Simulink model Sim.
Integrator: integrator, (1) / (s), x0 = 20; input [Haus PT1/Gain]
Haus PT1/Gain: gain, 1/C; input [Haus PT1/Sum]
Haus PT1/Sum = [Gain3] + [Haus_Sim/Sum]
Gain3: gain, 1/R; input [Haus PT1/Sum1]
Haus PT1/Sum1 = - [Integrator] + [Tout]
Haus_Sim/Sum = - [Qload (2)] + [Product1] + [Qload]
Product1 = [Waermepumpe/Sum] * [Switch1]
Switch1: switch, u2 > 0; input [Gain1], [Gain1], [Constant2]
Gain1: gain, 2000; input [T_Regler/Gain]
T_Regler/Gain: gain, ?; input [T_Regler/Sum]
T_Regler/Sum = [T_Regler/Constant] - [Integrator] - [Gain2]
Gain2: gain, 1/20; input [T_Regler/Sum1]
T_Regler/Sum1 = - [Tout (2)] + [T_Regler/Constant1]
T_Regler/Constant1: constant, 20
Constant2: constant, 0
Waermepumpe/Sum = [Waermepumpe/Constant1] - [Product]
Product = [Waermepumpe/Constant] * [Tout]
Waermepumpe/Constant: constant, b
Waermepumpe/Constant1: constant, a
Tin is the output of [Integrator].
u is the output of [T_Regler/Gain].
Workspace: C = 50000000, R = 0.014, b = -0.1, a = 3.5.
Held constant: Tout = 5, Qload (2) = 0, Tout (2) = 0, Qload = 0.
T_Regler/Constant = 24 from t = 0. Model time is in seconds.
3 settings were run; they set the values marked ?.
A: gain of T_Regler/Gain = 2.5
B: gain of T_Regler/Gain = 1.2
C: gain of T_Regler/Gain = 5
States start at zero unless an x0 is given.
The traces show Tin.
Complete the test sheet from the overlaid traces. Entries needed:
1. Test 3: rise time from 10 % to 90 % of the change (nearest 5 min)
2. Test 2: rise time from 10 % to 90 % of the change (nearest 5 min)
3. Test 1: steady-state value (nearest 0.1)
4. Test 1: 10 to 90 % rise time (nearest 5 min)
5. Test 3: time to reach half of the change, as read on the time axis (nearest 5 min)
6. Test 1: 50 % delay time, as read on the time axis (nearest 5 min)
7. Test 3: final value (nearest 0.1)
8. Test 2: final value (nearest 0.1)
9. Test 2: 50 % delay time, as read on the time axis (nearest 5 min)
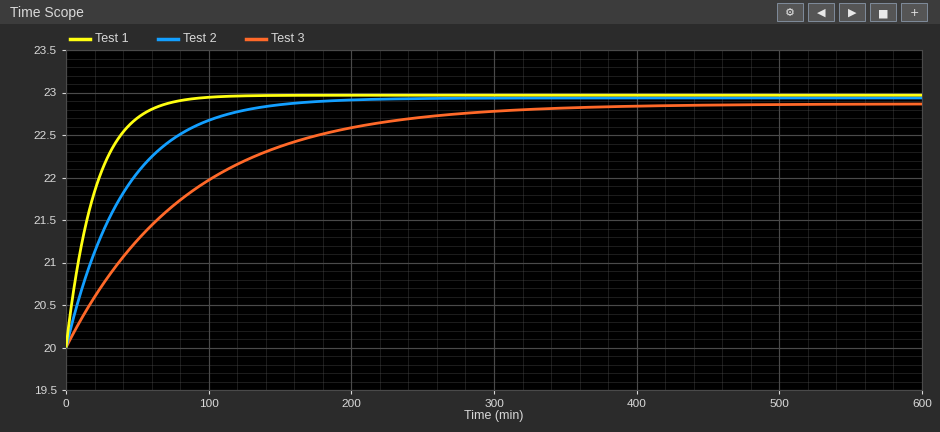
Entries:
190 min
90 min
23.0
45 min
60 min
15 min
22.9
22.9
30 min
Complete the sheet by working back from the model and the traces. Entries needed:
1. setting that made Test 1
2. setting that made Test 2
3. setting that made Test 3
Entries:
C
A
B
